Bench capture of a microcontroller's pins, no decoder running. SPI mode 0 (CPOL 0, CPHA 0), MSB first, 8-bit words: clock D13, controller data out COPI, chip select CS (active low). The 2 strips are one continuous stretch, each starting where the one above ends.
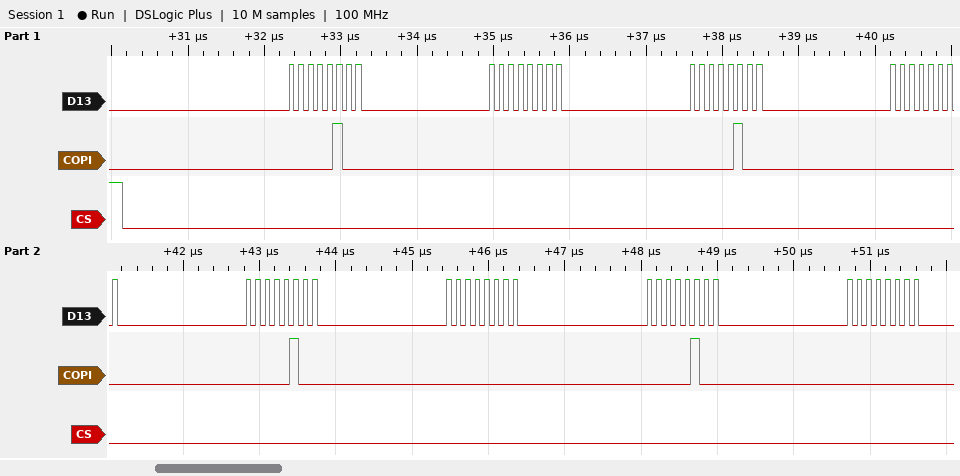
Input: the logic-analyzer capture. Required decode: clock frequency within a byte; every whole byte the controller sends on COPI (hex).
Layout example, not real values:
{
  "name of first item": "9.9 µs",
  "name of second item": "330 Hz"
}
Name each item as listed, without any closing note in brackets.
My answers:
{
  "clock frequency within a byte": "8 MHz",
  "every whole byte the controller sends on COPI": "04 00 04 00 04 00 04 00"
}
